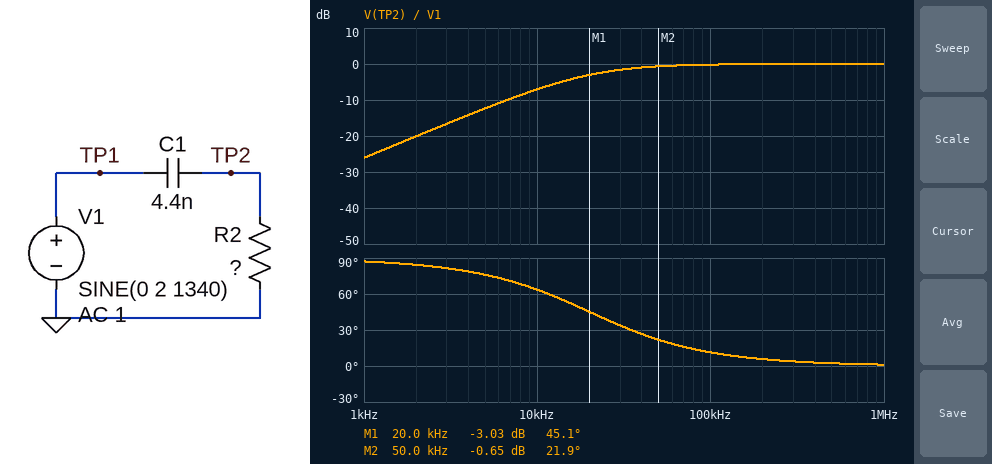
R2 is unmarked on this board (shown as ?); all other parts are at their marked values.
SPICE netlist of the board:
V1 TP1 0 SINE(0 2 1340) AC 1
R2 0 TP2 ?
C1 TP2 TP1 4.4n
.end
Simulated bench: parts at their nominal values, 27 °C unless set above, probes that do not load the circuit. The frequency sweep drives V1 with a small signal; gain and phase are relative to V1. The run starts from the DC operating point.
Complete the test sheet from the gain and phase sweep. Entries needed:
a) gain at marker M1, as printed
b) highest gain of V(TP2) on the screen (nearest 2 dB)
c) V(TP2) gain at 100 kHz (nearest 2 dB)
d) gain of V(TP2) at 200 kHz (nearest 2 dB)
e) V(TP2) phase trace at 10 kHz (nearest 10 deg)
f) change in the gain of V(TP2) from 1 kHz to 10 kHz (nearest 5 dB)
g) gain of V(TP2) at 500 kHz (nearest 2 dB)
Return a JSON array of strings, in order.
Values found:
["-3.03 dB", "0 dB", "0 dB", "0 dB", "60 deg", "20 dB", "0 dB"]
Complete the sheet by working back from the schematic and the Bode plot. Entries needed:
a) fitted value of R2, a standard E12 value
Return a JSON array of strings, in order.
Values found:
["1.8 kΩ"]
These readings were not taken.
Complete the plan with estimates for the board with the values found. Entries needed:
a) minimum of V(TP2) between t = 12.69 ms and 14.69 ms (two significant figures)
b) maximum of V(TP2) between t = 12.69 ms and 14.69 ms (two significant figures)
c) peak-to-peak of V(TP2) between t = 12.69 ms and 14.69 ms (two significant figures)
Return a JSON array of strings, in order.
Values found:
["-130 mV", "130 mV", "270 mV"]
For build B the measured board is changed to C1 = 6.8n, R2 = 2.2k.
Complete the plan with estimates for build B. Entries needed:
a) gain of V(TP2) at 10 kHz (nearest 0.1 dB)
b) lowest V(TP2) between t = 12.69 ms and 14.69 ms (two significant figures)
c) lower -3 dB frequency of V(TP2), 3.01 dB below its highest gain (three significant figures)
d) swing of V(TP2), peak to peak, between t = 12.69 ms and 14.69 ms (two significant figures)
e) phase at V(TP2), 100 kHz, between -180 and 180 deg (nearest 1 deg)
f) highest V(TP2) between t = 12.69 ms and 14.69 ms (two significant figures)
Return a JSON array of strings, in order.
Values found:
["-3.3 dB", "-250 mV", "10.6 kHz", "500 mV", "6 deg", "250 mV"]
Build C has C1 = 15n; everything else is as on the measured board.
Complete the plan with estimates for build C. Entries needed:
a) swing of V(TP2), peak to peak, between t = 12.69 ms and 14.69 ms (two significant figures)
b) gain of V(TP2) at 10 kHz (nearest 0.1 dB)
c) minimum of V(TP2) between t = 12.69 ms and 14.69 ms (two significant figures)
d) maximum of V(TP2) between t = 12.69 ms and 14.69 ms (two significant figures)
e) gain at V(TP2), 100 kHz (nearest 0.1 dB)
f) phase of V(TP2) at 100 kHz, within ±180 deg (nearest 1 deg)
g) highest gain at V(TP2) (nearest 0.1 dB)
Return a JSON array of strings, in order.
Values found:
["890 mV", "-1.3 dB", "-440 mV", "440 mV", "0 dB", "3 deg", "0 dB"]
